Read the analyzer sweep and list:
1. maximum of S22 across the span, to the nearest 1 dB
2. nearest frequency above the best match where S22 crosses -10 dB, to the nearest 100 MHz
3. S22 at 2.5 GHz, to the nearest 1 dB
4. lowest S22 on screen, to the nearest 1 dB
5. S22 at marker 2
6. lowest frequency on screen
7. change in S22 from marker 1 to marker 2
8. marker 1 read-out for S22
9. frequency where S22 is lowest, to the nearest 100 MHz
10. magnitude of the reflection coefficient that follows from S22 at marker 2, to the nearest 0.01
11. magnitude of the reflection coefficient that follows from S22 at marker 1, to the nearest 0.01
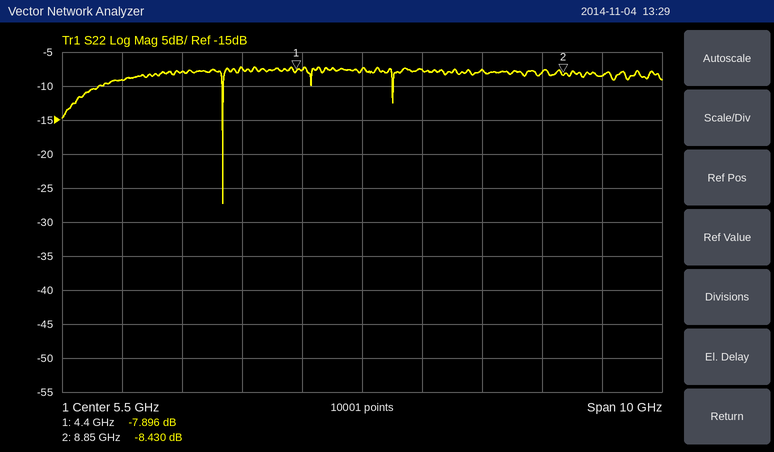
-7 dB
3.2 GHz
-8 dB
-27 dB
-8.430 dB
500 MHz
-0.534 dB
-7.896 dB
3.2 GHz
0.38
0.40
